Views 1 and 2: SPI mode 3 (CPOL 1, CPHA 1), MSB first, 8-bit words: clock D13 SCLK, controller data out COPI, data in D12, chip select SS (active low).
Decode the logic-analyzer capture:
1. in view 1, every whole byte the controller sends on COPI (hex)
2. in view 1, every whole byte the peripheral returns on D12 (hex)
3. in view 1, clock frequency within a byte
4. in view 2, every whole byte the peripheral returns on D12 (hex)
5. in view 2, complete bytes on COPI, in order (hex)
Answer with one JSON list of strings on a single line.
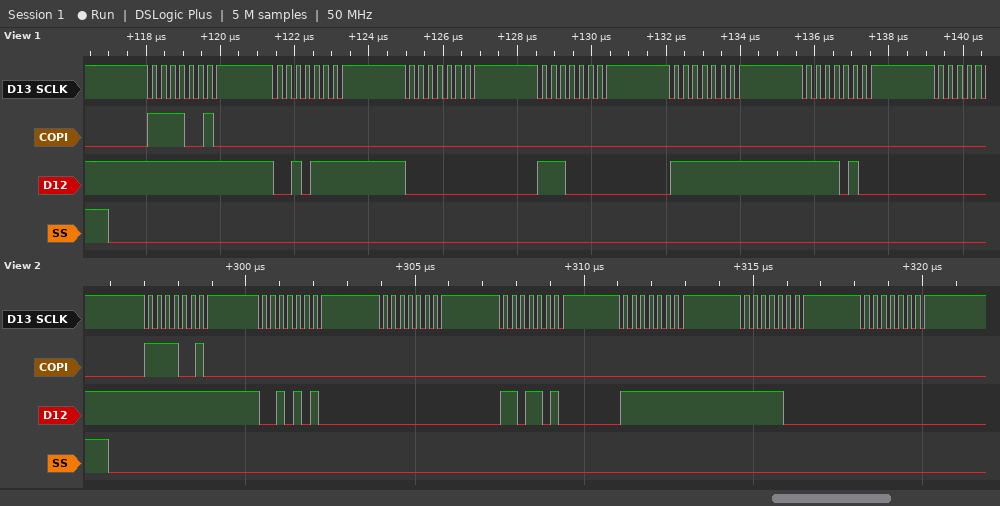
["0xF2 0x00 0x00 0x00 0x00 0x00", "0xFF 0x2F 0x00 0xE0 0xFF 0xF4", "4 MHz", "FF 2A 00 DA FF F8 00", "F2 00 00 00 00 00 00"]
